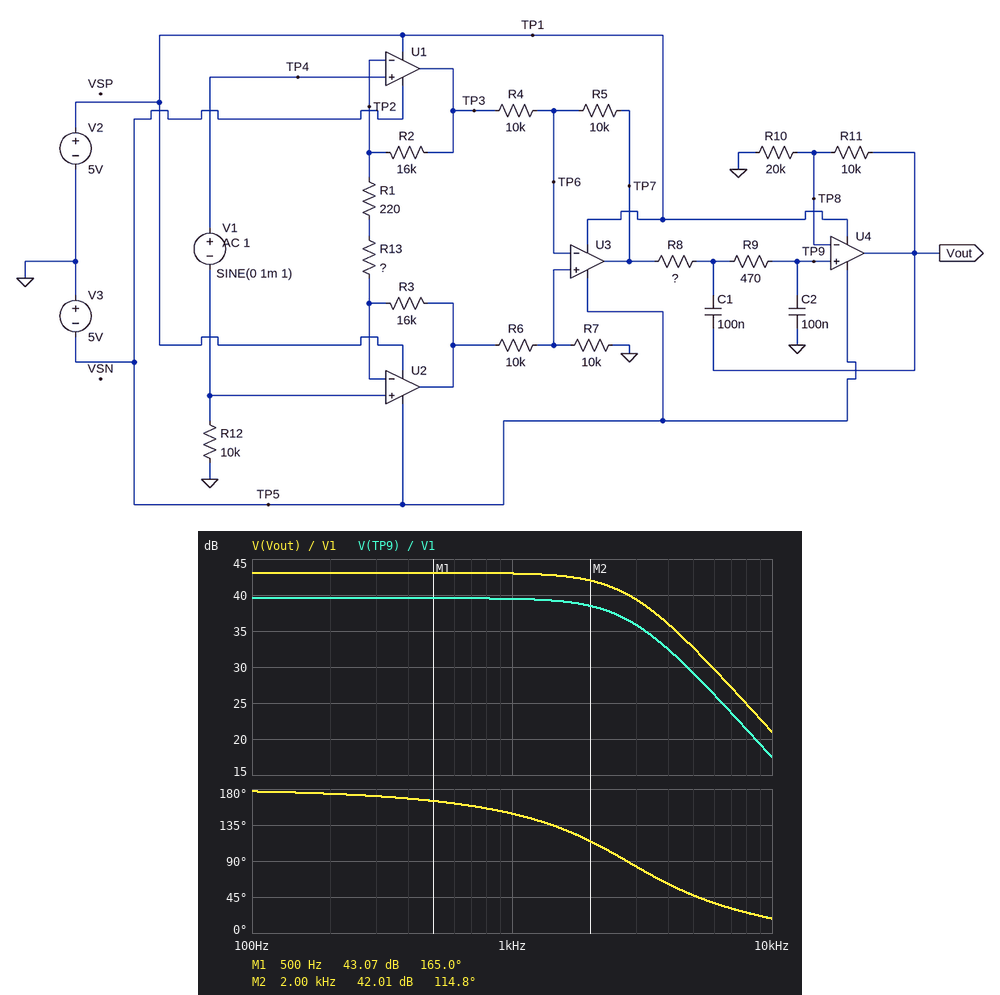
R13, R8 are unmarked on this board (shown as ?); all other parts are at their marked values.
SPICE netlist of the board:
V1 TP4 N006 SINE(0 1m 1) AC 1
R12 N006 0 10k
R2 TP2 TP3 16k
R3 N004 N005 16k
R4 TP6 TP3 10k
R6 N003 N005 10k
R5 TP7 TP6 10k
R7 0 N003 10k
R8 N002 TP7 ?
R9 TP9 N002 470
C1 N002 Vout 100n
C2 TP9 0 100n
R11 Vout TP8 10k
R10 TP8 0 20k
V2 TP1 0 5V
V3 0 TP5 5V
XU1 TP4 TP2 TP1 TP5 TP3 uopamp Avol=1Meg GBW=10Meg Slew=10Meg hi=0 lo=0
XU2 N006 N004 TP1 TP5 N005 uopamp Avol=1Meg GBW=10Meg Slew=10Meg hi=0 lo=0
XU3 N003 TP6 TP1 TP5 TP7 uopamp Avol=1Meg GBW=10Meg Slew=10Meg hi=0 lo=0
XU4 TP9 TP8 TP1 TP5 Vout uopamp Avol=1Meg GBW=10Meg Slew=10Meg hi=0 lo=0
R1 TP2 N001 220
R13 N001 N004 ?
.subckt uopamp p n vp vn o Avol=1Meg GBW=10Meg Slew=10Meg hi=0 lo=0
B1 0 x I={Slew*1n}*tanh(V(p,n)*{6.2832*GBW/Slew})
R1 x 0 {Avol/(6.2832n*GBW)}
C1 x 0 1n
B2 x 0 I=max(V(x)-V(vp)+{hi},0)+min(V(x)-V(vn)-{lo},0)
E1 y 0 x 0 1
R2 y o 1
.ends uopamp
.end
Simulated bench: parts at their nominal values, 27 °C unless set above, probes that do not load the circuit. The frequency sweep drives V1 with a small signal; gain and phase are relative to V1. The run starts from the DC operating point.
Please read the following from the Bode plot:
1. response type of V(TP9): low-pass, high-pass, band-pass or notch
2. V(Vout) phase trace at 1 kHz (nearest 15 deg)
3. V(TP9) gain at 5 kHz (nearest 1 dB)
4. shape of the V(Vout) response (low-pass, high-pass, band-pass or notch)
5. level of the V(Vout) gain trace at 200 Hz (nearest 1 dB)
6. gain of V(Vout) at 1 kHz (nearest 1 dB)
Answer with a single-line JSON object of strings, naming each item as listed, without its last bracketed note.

{"response type of V(TP9): low-pass, high-pass, band-pass or notch": "low-pass", "V(Vout) phase trace at 1 kHz": "150 deg", "V(TP9) gain at 5 kHz": "29 dB", "shape of the V(Vout) response": "low-pass", "level of the V(Vout) gain trace at 200 Hz": "43 dB", "gain of V(Vout) at 1 kHz": "43 dB"}
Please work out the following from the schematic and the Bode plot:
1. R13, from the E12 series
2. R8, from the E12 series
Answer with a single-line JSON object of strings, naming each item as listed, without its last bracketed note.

{"R13, from the E12 series": "120 Ω", "R8, from the E12 series": "680 Ω"}
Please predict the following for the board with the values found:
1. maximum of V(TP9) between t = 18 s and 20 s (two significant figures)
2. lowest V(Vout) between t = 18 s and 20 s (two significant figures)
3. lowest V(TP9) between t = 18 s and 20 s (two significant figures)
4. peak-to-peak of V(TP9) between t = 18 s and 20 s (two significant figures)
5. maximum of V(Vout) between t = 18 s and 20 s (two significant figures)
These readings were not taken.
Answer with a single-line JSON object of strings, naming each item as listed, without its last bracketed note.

{"maximum of V(TP9) between t = 18 s and 20 s": "95 mV", "lowest V(Vout) between t = 18 s and 20 s": "-140 mV", "lowest V(TP9) between t = 18 s and 20 s": "-95 mV", "peak-to-peak of V(TP9) between t = 18 s and 20 s": "190 mV", "maximum of V(Vout) between t = 18 s and 20 s": "140 mV"}
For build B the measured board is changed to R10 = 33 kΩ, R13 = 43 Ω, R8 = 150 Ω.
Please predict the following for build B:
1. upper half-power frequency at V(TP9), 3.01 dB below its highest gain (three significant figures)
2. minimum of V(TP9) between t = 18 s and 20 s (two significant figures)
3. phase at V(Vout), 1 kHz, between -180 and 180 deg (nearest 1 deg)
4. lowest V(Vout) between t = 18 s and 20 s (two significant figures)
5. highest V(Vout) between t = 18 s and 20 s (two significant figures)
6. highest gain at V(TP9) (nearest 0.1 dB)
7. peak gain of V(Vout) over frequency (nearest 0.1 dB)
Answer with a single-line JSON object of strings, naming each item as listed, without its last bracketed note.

{"upper half-power frequency at V(TP9), 3.01 dB below its highest gain": "3.45 kHz", "minimum of V(TP9) between t = 18 s and 20 s": "-120 mV", "phase at V(Vout), 1 kHz, between -180 and 180 deg": "159 deg", "lowest V(Vout) between t = 18 s and 20 s": "-160 mV", "highest V(Vout) between t = 18 s and 20 s": "160 mV", "highest gain at V(TP9)": "41.8 dB", "peak gain of V(Vout) over frequency": "44.1 dB"}
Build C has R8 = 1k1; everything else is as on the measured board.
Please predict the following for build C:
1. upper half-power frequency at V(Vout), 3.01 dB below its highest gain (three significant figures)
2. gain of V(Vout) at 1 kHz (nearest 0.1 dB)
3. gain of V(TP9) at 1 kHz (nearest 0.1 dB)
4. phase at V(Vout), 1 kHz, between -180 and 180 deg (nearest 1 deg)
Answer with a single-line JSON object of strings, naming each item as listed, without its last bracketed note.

{"upper half-power frequency at V(Vout), 3.01 dB below its highest gain": "2.21 kHz", "gain of V(Vout) at 1 kHz": "42.9 dB", "gain of V(TP9) at 1 kHz": "39.4 dB", "phase at V(Vout), 1 kHz, between -180 and 180 deg": "141 deg"}
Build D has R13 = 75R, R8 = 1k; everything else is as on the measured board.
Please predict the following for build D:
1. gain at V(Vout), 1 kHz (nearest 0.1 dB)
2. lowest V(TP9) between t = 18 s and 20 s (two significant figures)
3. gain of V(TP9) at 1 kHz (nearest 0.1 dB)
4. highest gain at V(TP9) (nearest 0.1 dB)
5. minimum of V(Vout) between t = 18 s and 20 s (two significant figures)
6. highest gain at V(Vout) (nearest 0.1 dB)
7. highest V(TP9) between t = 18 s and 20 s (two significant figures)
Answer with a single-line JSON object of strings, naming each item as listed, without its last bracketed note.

{"gain at V(Vout), 1 kHz": "44.2 dB", "lowest V(TP9) between t = 18 s and 20 s": "-110 mV", "gain of V(TP9) at 1 kHz": "40.6 dB", "highest gain at V(TP9)": "40.8 dB", "minimum of V(Vout) between t = 18 s and 20 s": "-160 mV", "highest gain at V(Vout)": "44.3 dB", "highest V(TP9) between t = 18 s and 20 s": "110 mV"}
